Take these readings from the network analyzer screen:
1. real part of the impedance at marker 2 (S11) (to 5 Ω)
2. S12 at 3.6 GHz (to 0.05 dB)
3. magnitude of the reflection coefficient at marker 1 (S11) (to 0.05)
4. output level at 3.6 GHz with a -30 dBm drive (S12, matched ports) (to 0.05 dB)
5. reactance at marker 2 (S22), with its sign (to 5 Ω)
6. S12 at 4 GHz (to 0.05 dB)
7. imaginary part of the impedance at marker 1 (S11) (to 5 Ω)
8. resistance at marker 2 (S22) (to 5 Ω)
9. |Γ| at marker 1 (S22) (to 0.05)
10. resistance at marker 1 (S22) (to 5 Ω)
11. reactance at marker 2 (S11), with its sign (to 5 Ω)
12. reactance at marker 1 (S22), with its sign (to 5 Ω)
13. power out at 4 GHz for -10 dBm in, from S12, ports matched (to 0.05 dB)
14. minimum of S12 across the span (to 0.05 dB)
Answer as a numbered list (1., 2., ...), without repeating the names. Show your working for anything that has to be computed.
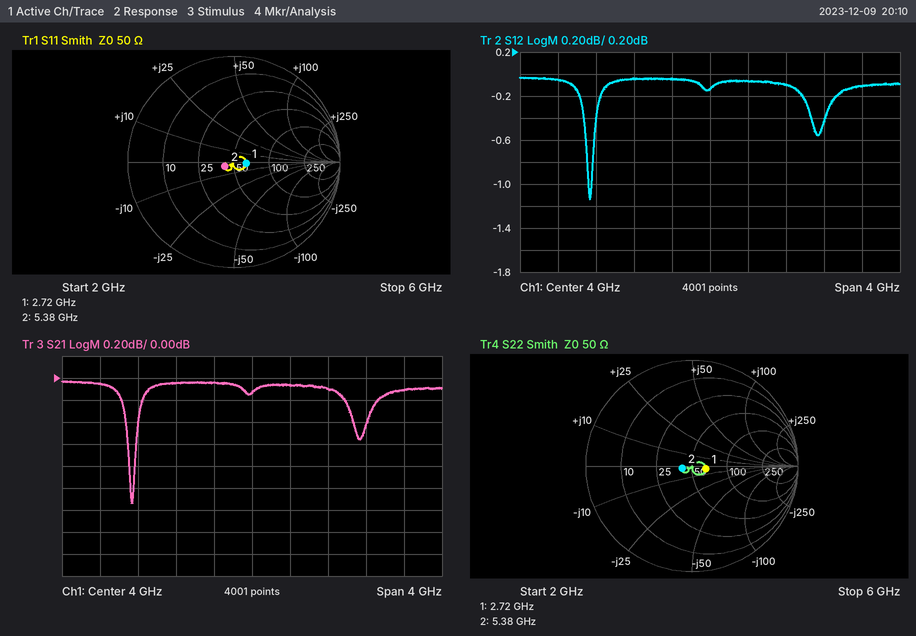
1. 40 Ω
2. -0.05 dB
3. 0.10
4. -30 dBm + (-0.05 dB) = -30.05 dBm
5. 0 Ω
6. -0.15 dB
7. 0 Ω
8. 40 Ω
9. 0.15
10. 65 Ω
11. -5 Ω
12. -5 Ω
13. -10 dBm + (-0.15 dB) = -10.15 dBm
14. -1.15 dB
